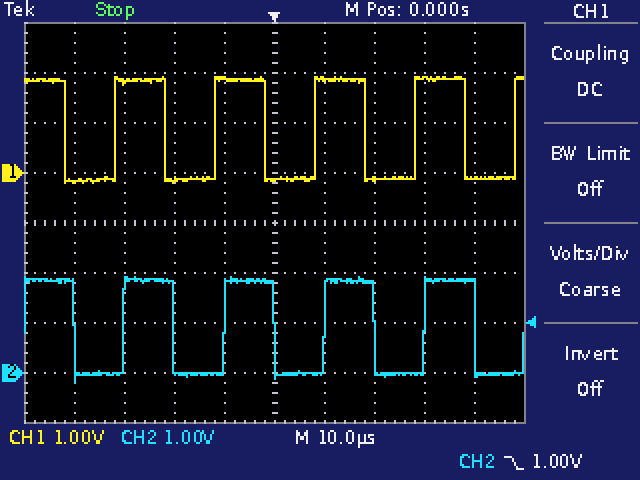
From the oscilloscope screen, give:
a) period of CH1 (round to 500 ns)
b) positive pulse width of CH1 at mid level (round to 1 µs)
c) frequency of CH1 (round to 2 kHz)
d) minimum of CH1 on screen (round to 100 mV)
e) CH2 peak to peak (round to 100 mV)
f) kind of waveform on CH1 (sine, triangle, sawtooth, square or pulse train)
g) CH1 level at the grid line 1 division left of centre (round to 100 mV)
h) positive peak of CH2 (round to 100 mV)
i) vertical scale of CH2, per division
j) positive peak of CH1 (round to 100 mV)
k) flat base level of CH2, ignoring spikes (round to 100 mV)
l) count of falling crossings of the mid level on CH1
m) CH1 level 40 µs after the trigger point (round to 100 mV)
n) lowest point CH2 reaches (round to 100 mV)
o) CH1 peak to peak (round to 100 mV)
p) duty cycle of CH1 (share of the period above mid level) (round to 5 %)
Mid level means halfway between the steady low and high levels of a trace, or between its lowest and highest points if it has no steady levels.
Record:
20.0 µs
10 µs
50 kHz
-200 mV
2.1 V
square
1.9 V
1.9 V
1 V
1.9 V
0.0 V
5
-100 mV
-200 mV
2.1 V
50 %
